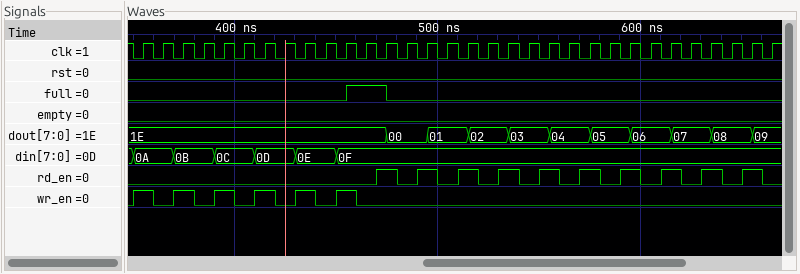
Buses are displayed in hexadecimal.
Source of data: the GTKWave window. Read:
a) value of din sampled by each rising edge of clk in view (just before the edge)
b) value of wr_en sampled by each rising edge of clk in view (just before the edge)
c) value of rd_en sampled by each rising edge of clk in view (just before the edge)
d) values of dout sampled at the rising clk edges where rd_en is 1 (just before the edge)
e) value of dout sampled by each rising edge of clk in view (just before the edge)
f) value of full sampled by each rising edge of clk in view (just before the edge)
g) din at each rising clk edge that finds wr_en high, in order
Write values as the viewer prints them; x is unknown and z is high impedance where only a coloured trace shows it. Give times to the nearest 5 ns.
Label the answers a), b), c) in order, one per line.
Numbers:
a) 0A, 0A, 0B, 0B, 0C, 0C, 0D, 0D, 0E, 0E, 0F, 0F, 0F, 0F, 0F, 0F, 0F, 0F, 0F, 0F, 0F, 0F, 0F, 0F, 0F, 0F, 0F, 0F, 0F, 0F, 0F, 0F
b) 1 0 1 0 1 0 1 0 1 0 1 0 0 0 0 0 0 0 0 0 0 0 0 0 0 0 0 0 0 0 0 0
c) 0 0 0 0 0 0 0 0 0 0 0 0 1 0 1 0 1 0 1 0 1 0 1 0 1 0 1 0 1 0 1 0
d) 1E, 00, 01, 02, 03, 04, 05, 06, 07, 08
e) 1E, 1E, 1E, 1E, 1E, 1E, 1E, 1E, 1E, 1E, 1E, 1E, 1E, 00, 00, 01, 01, 02, 02, 03, 03, 04, 04, 05, 05, 06, 06, 07, 07, 08, 08, 09
f) 0 0 0 0 0 0 0 0 0 0 0 1 1 0 0 0 0 0 0 0 0 0 0 0 0 0 0 0 0 0 0 0
g) 0A, 0B, 0C, 0D, 0E, 0F
